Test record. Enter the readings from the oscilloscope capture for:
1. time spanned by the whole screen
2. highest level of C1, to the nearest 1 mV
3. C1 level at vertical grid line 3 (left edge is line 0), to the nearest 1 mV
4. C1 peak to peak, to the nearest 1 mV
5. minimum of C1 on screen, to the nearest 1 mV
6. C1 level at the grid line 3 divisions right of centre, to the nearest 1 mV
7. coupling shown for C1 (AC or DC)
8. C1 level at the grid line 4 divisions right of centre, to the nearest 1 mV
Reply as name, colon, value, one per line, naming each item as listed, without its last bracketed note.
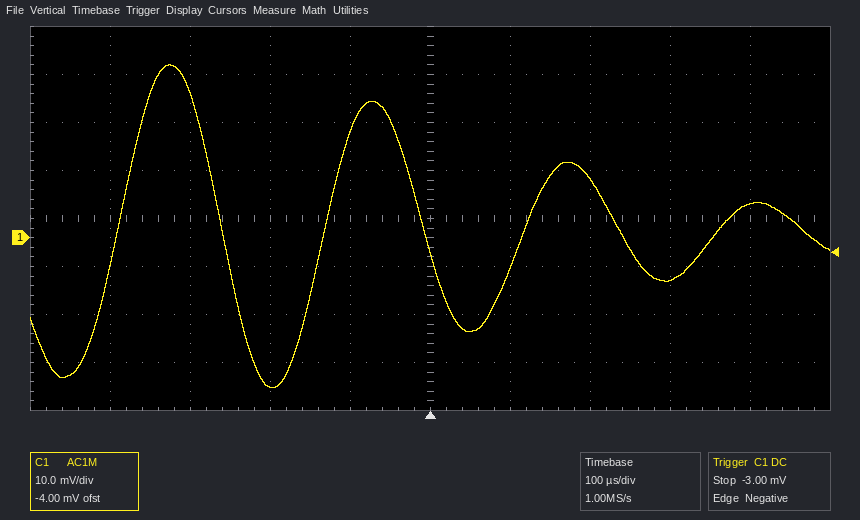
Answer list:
time spanned by the whole screen: 1 ms
highest level of C1, to the nearest 1 mV: 36 mV
C1 level at vertical grid line 3 (left edge is line 0), to the nearest 1 mV: -31 mV
C1 peak to peak, to the nearest 1 mV: 67 mV
minimum of C1 on screen, to the nearest 1 mV: -31 mV
C1 level at the grid line 3 divisions right of centre, to the nearest 1 mV: -9 mV
coupling shown for C1: AC
C1 level at the grid line 4 divisions right of centre, to the nearest 1 mV: 7 mV
